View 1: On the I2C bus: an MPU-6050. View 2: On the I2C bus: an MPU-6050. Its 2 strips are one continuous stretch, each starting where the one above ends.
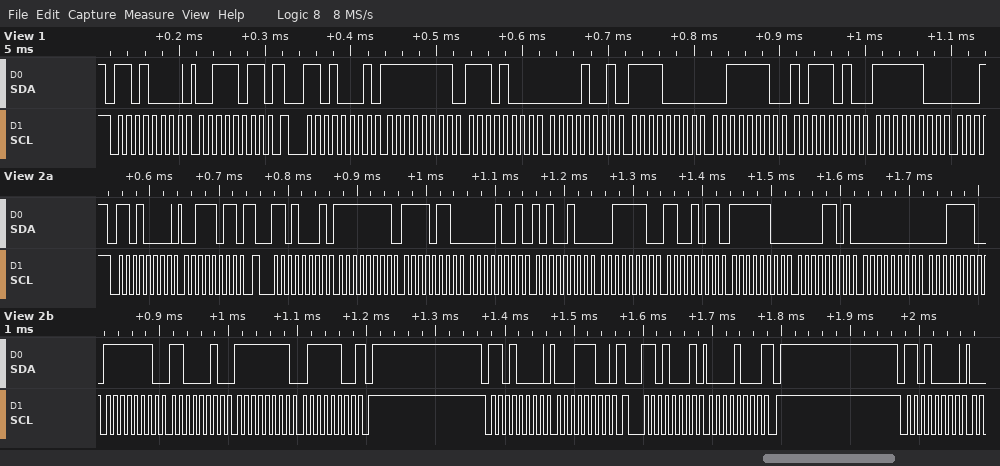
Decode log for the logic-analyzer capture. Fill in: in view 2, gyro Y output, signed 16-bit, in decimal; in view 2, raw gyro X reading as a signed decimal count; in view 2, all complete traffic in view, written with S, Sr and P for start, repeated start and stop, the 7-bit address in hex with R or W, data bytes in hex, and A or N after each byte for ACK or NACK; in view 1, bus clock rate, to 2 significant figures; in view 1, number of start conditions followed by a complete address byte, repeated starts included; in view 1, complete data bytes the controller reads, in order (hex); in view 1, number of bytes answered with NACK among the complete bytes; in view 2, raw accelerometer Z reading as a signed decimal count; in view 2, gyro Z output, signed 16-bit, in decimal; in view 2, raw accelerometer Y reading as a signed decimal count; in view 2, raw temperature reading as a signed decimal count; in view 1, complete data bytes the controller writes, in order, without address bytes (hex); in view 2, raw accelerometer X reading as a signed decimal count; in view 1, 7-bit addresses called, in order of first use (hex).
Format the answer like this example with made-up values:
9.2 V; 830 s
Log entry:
-318; 30; S 68W A 3B A Sr 68R A FF A F6 A 09 A A4 A 3E A CB A FC A 0D A 00 A 1E A FE A C2 A FF A 7C N P S 68W A 1C A Sr 68R A 08 N P S 68W A; 100 kHz; 2; FF E8 09 F0 3E BA FC; 0; 16075; -132; 2468; -1011; 3B; -10; 0x68
